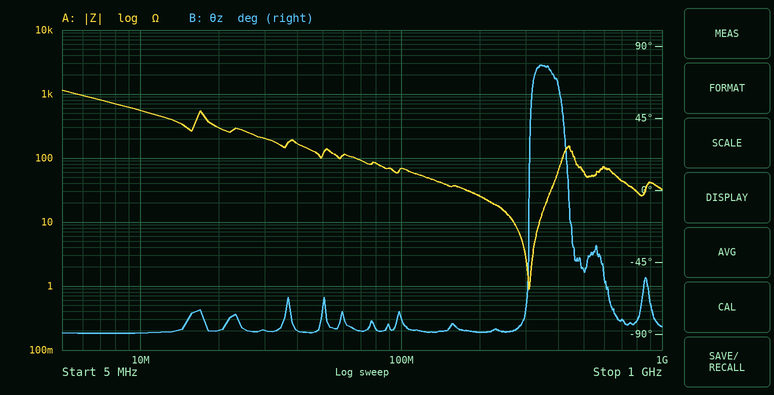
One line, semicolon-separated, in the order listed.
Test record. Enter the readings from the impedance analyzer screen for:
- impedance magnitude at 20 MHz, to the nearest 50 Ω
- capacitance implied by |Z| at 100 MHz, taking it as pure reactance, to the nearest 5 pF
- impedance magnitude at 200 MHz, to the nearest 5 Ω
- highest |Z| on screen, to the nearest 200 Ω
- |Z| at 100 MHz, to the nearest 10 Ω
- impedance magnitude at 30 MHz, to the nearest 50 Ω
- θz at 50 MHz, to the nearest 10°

300 Ω; 25 pF; 25 Ω; 1.2 kΩ; 70 Ω; 200 Ω; -70°
